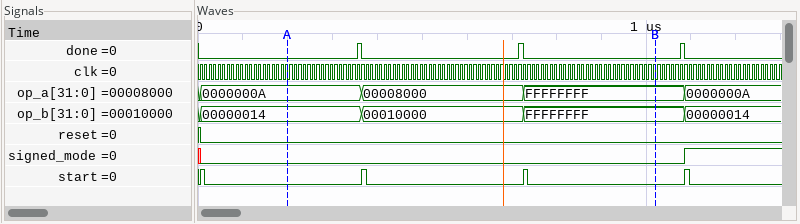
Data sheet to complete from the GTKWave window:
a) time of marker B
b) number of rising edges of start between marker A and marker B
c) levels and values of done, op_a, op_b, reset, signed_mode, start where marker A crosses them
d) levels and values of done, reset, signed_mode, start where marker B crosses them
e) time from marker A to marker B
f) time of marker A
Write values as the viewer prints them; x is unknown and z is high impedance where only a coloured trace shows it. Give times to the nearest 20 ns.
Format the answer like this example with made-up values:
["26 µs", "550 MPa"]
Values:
["1020 ns", "2", "done=0, op_a=0000000A, op_b=00000014, reset=0, signed_mode=0, start=0", "done=0, reset=0, signed_mode=0, start=0", "820 ns", "200 ns"]
